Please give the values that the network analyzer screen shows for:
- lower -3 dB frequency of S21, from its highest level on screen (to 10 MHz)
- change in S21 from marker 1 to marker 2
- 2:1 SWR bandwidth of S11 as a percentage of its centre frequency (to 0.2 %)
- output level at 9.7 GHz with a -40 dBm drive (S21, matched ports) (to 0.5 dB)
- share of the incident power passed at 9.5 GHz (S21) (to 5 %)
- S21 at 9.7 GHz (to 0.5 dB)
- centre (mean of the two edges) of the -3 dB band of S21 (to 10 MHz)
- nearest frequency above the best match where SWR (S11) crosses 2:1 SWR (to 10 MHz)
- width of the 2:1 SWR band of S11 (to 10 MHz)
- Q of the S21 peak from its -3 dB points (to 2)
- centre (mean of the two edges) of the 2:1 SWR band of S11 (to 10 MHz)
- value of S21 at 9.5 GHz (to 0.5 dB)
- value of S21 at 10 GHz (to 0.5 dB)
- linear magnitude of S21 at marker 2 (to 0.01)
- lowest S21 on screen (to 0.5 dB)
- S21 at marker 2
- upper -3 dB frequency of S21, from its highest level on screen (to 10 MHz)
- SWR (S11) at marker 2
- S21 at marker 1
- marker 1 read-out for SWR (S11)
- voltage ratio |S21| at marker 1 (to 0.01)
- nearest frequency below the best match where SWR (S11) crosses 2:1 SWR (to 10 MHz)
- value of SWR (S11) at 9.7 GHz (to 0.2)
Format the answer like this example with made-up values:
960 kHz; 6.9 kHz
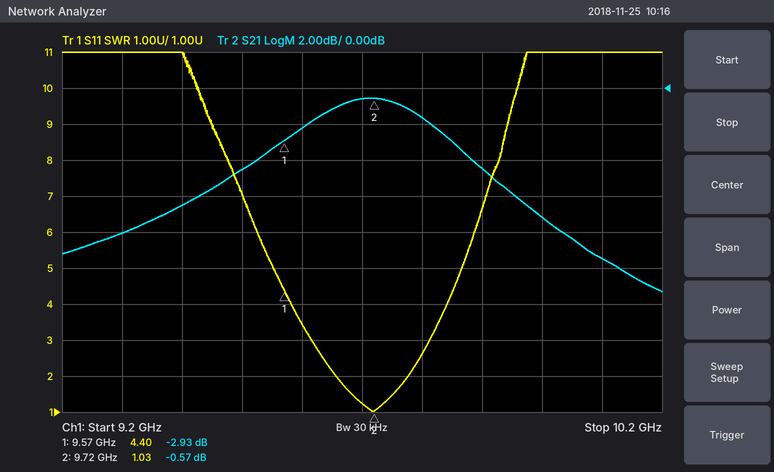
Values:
9.54 GHz; 2.36 dB; 1.2 %; -40.5 dBm; 35 %; -0.5 dB; 9.71 GHz; 9.78 GHz; 120 MHz; 30; 9.72 GHz; -4.5 dB; -7.0 dB; 0.94; -11.5 dB; -0.57 dB; 9.87 GHz; 1.03; -2.93 dB; 4.40; 0.71; 9.66 GHz; 1.2
